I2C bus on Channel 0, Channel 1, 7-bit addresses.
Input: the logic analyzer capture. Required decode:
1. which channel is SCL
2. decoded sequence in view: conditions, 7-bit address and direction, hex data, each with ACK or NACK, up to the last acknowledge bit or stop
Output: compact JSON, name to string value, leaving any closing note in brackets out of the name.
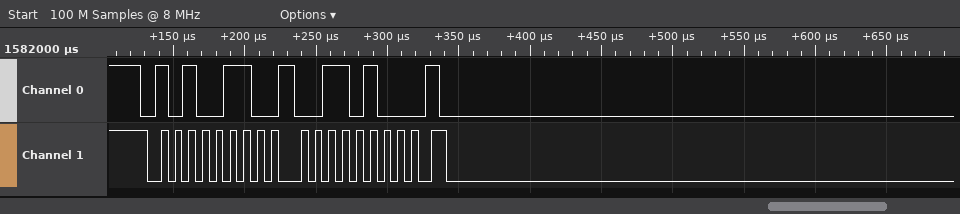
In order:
{"which channel is SCL": "Channel 1", "decoded sequence in view: conditions, 7-bit address and direction, hex data, each with ACK or NACK, up to the last acknowledge bit or stop": "start, address 53 write ACK, 34 ACK"}
